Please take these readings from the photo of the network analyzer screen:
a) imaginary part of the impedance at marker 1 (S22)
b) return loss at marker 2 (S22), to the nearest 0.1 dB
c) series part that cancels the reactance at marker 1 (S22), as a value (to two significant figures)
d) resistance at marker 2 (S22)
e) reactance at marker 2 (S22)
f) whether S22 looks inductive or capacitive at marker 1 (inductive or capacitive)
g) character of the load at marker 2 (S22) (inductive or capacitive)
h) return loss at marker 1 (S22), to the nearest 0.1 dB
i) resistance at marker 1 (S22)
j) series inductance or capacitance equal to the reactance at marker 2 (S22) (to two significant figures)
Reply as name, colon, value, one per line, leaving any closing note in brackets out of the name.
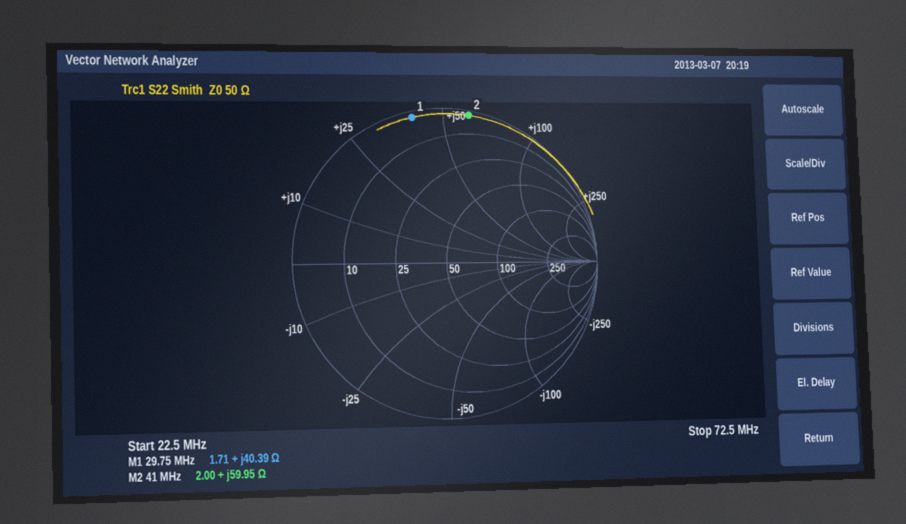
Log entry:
imaginary part of the impedance at marker 1: +40.39 Ω
return loss at marker 2 (S22), to the nearest 0.1 dB: 0.3 dB
series part that cancels the reactance at marker 1 (S22), as a value: 130 pF
resistance at marker 2: 2.00 Ω
reactance at marker 2: +59.95 Ω
whether S22 looks inductive or capacitive at marker 1: inductive
character of the load at marker 2 (S22): inductive
return loss at marker 1 (S22), to the nearest 0.1 dB: 0.4 dB
resistance at marker 1: 1.71 Ω
series inductance or capacitance equal to the reactance at marker 2 (S22): 230 nH
